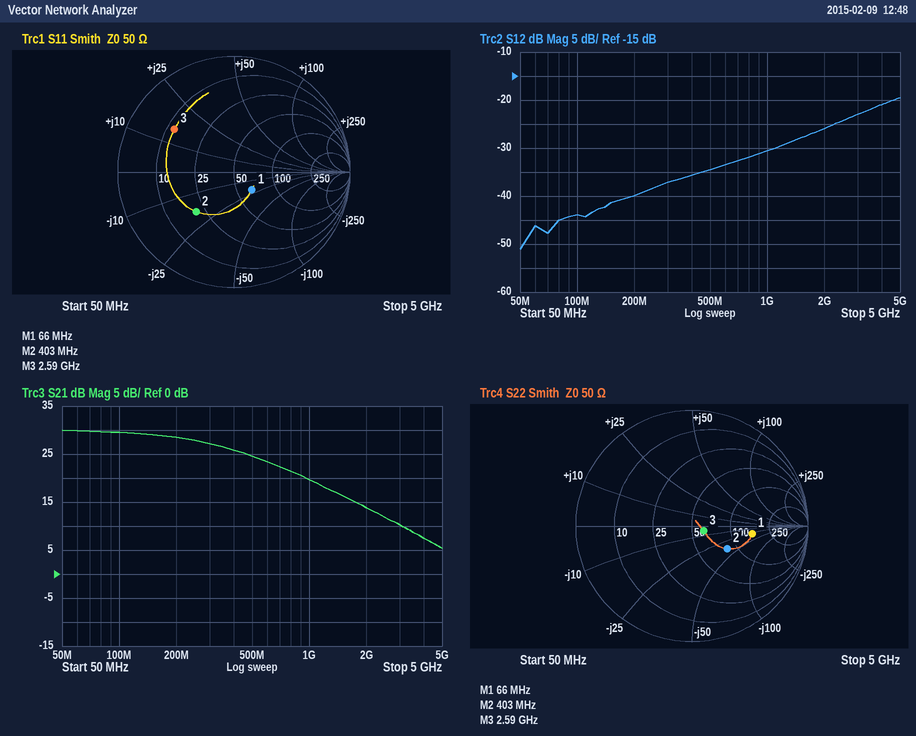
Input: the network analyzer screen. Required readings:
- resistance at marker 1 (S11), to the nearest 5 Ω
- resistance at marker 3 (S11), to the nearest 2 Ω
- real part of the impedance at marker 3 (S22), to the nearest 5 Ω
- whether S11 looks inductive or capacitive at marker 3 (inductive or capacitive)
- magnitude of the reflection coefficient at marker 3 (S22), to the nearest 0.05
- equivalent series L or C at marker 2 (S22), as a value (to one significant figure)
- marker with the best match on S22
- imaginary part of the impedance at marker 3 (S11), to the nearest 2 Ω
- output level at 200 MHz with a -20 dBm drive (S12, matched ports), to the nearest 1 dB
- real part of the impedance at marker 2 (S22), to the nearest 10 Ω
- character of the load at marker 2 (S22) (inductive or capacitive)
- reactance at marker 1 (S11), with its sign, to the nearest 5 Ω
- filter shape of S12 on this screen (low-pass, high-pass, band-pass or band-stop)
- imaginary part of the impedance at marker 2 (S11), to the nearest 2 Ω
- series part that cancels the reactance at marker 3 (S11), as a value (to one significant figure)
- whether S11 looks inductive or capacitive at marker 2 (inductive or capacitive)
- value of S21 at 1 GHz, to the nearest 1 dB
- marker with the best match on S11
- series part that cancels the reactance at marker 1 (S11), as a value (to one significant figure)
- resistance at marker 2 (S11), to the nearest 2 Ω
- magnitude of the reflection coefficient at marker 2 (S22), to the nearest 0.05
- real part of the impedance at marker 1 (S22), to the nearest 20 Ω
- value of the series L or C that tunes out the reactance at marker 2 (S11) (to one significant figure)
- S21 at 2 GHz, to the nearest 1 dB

65 Ω
12 Ω
60 Ω
inductive
0.10
10 pF
marker 3
+16 Ω
-60 dBm
80 Ω
capacitive
-20 Ω
high-pass
-18 Ω
4 pF
capacitive
20 dB
marker 1
50 nH
20 Ω
0.35
160 Ω
7 nH
14 dB
